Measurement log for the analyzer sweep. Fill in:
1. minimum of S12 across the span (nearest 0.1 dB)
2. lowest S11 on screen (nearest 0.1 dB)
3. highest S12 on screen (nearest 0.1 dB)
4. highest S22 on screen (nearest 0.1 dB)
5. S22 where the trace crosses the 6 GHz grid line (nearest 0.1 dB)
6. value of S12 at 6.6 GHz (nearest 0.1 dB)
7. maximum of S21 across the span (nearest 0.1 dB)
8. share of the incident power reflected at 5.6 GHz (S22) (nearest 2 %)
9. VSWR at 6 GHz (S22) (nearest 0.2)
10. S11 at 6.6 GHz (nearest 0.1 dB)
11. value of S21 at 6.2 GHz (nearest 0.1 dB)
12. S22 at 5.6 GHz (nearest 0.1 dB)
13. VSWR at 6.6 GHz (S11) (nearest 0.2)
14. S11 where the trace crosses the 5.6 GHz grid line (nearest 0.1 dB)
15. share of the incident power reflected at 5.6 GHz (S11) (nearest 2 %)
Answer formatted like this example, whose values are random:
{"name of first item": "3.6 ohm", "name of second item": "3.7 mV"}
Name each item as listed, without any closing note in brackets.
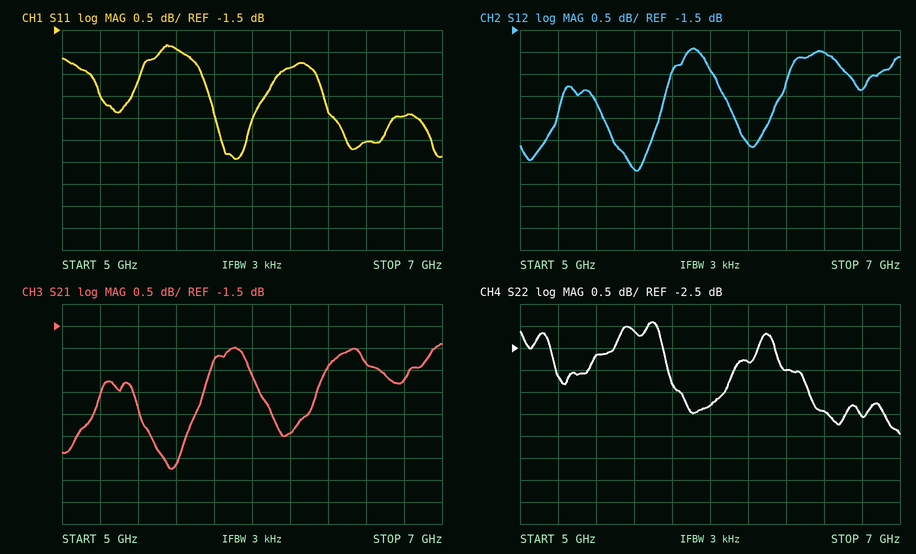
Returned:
{"minimum of S12 across the span": "-4.7 dB", "lowest S11 on screen": "-4.4 dB", "highest S12 on screen": "-1.9 dB", "highest S22 on screen": "-1.9 dB", "S22 where the trace crosses the 6 GHz grid line": "-3.8 dB", "value of S12 at 6.6 GHz": "-2.0 dB", "maximum of S21 across the span": "-1.9 dB", "share of the incident power reflected at 5.6 GHz (S22)": "62 %", "VSWR at 6 GHz (S22)": "4.6", "S11 at 6.6 GHz": "-4.0 dB", "value of S21 at 6.2 GHz": "-3.9 dB", "S22 at 5.6 GHz": "-2.1 dB", "VSWR at 6.6 GHz (S11)": "4.4", "S11 where the trace crosses the 5.6 GHz grid line": "-1.9 dB", "share of the incident power reflected at 5.6 GHz (S11)": "64 %"}
